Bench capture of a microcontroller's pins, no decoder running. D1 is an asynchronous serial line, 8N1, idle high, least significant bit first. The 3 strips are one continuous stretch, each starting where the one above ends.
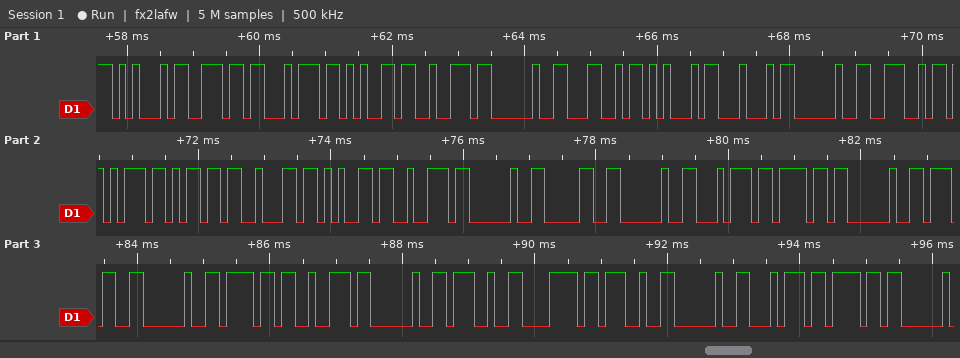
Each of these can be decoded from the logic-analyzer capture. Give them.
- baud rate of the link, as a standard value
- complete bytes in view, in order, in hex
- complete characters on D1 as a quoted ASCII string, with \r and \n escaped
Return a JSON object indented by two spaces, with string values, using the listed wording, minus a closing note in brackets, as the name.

{
  "baud rate of the link, as a standard value": "9600 baud",
  "complete bytes in view, in order, in hex": "45 6E 74 65 72 20 4C 45 44 20 4E 75 6D 62 65 72 20 30 20 74 6F 20 37 20 6F 72 20 27 78 27 20 74 6F",
  "complete characters on D1 as a quoted ASCII string, with \\r and \\n escaped": "\"Enter LED Number 0 to 7 or 'x' to\""
}
